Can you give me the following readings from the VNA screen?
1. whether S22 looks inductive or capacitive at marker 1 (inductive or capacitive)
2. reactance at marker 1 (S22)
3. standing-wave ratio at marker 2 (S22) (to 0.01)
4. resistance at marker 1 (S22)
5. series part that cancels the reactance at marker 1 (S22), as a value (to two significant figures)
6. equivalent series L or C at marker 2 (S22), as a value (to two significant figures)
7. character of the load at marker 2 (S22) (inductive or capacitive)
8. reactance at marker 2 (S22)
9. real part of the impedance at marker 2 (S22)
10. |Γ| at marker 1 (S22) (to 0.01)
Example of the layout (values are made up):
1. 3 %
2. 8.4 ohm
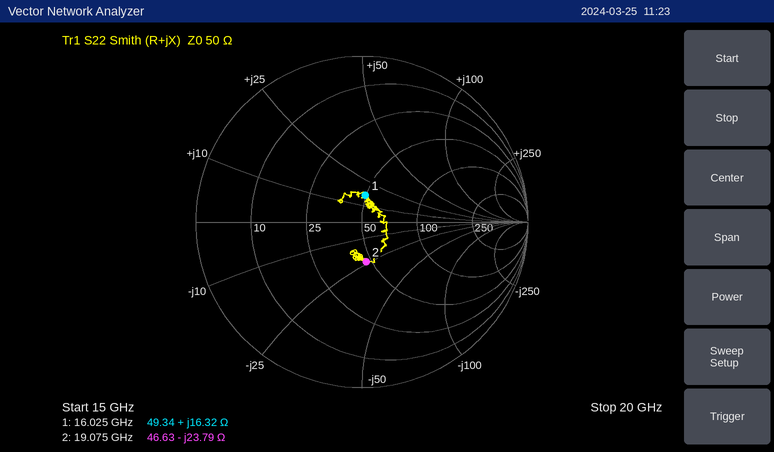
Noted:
1. inductive
2. +16.32 Ω
3. 1.64
4. 49.34 Ω
5. 610 fF
6. 350 fF
7. capacitive
8. -23.79 Ω
9. 46.63 Ω
10. 0.16
